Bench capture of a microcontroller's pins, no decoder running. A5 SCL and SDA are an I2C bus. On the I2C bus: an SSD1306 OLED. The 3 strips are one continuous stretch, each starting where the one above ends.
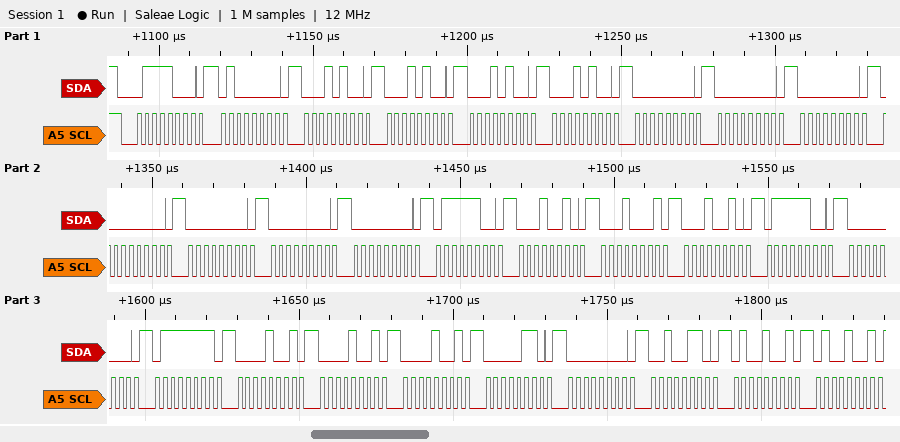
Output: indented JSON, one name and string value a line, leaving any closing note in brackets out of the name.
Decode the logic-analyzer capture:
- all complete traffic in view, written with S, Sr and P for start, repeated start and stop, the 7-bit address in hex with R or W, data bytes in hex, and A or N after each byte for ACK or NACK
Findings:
{
  "all complete traffic in view, written with S, Sr and P for start, repeated start and stop, the 7-bit address in hex with R or W, data bytes in hex, and A or N after each byte for ACK or NACK": "S 3CW A 40 A 14 A 14 A 14 A 14 A 00 A 00 A 00 A 00 A 00 A 00 A 00 A 7C A 12 A 11 A 12 A 7C A 00 A 7F A 09 A 09 A 09 A 06 A 00 A 26 A 49 A 49 A"
}
